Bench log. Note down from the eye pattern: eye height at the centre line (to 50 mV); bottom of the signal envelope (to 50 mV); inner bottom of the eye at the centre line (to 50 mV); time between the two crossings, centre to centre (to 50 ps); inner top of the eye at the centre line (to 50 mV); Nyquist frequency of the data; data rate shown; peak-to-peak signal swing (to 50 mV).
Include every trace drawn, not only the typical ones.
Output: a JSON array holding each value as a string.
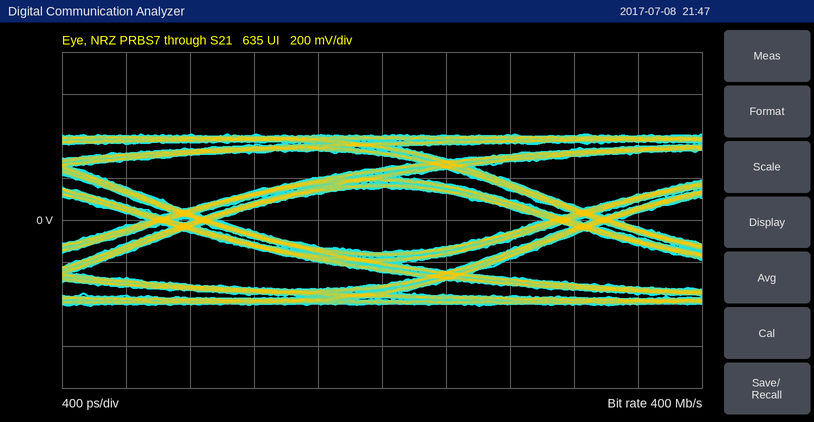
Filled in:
["300 mV", "-400 mV", "-150 mV", "2.50 ns", "150 mV", "200 MHz", "400 Mb/s", "800 mV"]
